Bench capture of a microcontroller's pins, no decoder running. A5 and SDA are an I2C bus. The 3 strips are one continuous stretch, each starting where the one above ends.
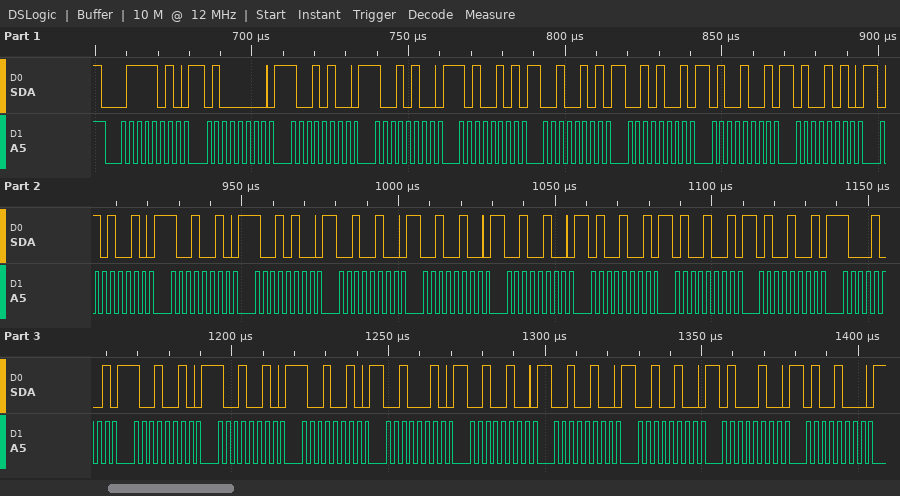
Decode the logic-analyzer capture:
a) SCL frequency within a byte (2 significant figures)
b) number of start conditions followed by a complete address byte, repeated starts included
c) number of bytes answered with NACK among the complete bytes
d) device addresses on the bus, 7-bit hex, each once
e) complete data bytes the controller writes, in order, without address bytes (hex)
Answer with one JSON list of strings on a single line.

["400 kHz", "1", "0", "0x3D", "40 94 94 A5 25 29 49 4A 52 92 94 24 24 24 49 49 49 89 92 92 92 22 24 24 24 44 48"]
